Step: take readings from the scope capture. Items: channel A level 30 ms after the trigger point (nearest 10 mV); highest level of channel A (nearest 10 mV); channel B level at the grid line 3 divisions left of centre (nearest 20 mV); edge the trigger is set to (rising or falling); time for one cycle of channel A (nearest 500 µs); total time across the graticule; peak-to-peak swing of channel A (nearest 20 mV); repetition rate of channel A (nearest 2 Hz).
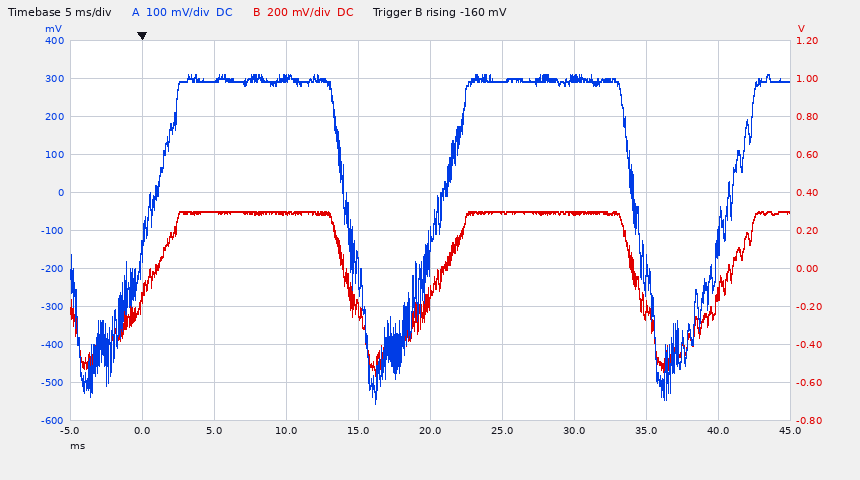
300 mV
310 mV
300 mV
rising
20.0 ms
50 ms
860 mV
50 Hz
